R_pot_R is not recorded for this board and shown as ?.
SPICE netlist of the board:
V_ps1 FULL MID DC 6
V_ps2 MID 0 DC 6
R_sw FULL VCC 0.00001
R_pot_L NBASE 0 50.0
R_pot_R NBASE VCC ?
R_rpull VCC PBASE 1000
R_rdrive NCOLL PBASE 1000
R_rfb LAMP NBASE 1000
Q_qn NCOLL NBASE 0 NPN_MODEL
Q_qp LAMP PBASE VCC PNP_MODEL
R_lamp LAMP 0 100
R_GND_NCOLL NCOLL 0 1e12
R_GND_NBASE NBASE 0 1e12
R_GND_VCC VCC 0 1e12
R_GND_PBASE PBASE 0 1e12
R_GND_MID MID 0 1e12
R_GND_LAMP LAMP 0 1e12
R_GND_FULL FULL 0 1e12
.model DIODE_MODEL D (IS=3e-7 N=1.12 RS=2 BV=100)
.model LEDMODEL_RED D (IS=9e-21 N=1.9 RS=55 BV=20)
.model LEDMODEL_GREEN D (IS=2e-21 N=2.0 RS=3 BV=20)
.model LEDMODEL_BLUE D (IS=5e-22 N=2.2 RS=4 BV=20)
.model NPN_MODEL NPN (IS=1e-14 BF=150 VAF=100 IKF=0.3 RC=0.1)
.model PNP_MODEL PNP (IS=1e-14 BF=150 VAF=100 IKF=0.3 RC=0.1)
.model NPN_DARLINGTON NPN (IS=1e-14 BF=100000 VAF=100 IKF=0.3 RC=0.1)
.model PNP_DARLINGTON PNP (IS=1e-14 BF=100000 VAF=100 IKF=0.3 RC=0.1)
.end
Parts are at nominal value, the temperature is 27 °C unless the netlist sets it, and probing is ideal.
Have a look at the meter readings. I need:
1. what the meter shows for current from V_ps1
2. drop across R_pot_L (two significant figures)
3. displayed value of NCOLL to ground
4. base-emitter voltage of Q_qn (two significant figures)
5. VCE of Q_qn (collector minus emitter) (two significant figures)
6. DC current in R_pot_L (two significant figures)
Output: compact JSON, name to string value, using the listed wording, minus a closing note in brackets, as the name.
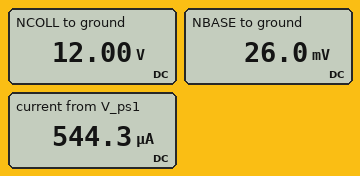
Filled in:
{"what the meter shows for current from V_ps1": "544.3 µA", "drop across R_pot_L": "26 mV", "displayed value of NCOLL to ground": "12.00 V", "base-emitter voltage of Q_qn": "26 mV", "VCE of Q_qn (collector minus emitter)": "12 V", "DC current in R_pot_L": "520 µA"}
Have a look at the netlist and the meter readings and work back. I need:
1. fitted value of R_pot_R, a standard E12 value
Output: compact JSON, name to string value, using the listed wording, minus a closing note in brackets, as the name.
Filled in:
{"fitted value of R_pot_R, a standard E12 value": "22 kΩ"}
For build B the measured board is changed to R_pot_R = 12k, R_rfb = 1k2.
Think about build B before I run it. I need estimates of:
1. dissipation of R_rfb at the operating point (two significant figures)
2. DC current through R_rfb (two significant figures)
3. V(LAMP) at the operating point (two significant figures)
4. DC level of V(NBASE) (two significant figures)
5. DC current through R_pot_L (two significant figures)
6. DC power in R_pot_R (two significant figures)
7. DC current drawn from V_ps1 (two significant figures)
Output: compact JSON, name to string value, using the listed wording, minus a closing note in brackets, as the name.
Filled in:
{"dissipation of R_rfb at the operating point": "1.6 µW", "DC current through R_rfb": "37 µA", "V(LAMP) at the operating point": "3.7 mV", "DC level of V(NBASE)": "48 mV", "DC current through R_pot_L": "960 µA", "DC power in R_pot_R": "12 mW", "DC current drawn from V_ps1": "1.0 mA"}
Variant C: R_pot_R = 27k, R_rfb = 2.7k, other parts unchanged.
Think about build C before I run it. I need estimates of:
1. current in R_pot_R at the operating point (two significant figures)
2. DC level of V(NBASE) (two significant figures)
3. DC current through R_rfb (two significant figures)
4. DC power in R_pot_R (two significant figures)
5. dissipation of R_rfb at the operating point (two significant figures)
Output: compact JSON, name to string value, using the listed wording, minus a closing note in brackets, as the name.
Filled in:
{"current in R_pot_R at the operating point": "440 µA", "DC level of V(NBASE)": "22 mV", "DC current through R_rfb": "7.8 µA", "DC power in R_pot_R": "5.3 mW", "dissipation of R_rfb at the operating point": "160 nW"}
